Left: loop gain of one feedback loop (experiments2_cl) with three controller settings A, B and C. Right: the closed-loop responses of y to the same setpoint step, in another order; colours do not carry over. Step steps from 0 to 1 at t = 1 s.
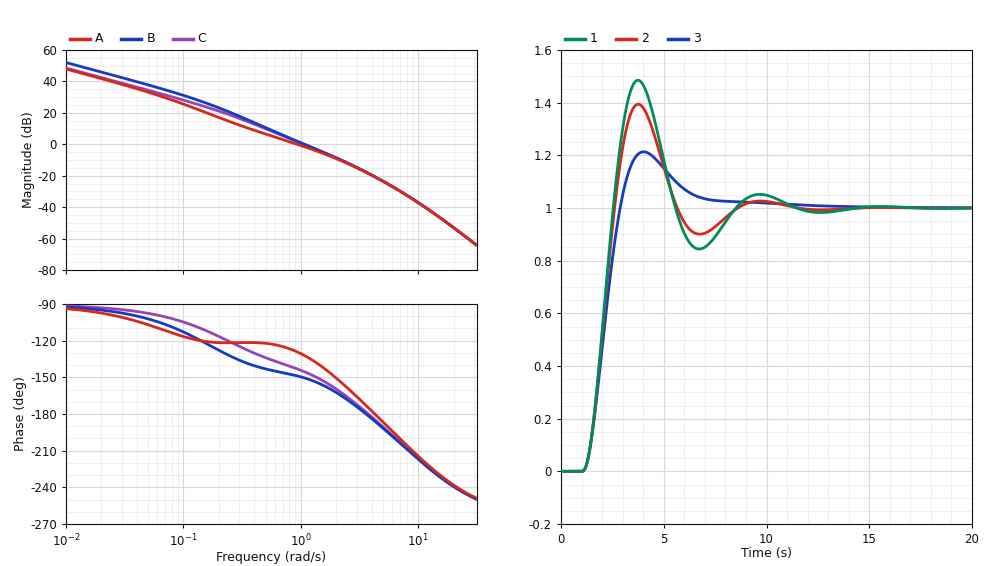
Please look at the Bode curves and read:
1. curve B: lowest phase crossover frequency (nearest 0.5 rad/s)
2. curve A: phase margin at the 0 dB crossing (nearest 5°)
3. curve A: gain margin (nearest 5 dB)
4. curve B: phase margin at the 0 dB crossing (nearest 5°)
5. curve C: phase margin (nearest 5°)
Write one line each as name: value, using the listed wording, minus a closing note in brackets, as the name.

curve B: lowest phase crossover frequency: 3.5 rad/s
curve A: phase margin at the 0 dB crossing: 50°
curve A: gain margin: 20 dB
curve B: phase margin at the 0 dB crossing: 30°
curve C: phase margin: 35°
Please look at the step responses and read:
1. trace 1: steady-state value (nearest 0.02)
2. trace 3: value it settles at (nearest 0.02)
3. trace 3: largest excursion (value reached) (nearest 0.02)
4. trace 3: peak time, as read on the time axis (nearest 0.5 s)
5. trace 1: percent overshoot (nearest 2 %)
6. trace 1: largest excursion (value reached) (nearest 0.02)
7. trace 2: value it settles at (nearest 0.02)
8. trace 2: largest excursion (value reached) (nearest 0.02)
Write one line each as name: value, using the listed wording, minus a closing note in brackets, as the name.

trace 1: steady-state value: 1.00
trace 3: value it settles at: 1.00
trace 3: largest excursion (value reached): 1.22
trace 3: peak time, as read on the time axis: 4.0 s
trace 1: percent overshoot: 48 %
trace 1: largest excursion (value reached): 1.48
trace 2: value it settles at: 1.00
trace 2: largest excursion (value reached): 1.40
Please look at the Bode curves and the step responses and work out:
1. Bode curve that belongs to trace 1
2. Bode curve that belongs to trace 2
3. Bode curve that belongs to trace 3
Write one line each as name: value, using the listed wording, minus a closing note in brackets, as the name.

Bode curve that belongs to trace 1: B
Bode curve that belongs to trace 2: C
Bode curve that belongs to trace 3: A
